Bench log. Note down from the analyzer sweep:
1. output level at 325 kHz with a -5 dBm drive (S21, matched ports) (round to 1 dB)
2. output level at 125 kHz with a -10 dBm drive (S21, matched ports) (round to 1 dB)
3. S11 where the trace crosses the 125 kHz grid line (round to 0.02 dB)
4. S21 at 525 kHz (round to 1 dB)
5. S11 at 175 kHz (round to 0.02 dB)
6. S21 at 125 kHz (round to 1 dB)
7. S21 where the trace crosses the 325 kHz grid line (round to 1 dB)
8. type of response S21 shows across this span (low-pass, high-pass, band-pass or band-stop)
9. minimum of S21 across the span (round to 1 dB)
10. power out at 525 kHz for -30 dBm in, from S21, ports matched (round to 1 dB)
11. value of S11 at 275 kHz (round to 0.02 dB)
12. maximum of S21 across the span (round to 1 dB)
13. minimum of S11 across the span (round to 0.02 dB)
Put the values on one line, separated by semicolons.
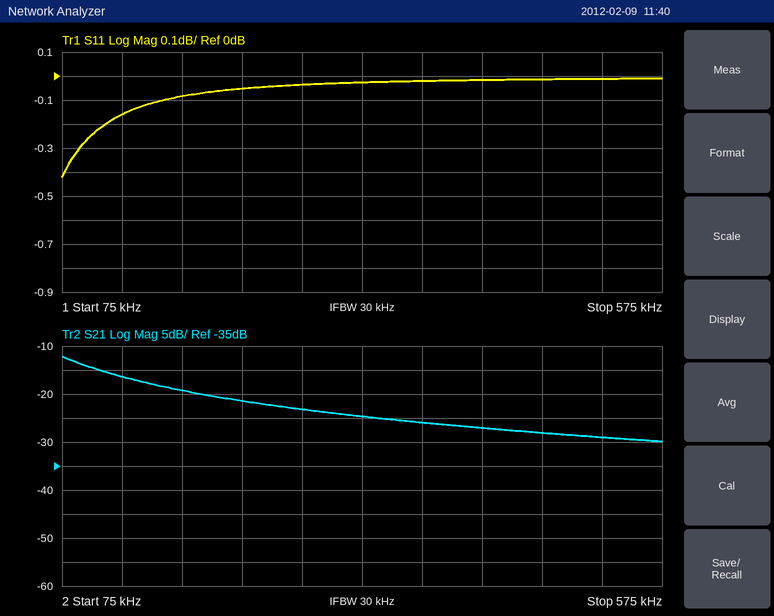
-30 dBm; -26 dBm; -0.16 dB; -29 dB; -0.08 dB; -16 dB; -25 dB; low-pass; -30 dB; -59 dBm; -0.04 dB; -12 dB; -0.42 dB
